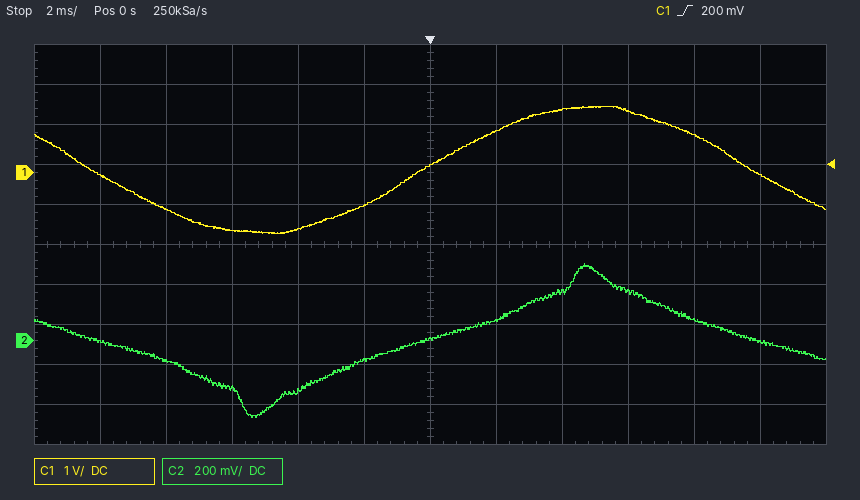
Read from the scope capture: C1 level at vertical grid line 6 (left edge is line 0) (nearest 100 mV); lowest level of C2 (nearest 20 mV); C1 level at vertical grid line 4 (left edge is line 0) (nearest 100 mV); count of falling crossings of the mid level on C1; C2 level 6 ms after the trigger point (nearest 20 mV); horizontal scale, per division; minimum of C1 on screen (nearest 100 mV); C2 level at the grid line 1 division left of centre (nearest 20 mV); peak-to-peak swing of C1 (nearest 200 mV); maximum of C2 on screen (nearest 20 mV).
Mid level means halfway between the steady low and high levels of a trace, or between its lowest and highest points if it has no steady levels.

200 mV
-380 mV
-1.4 V
2
240 mV
2 ms
-1.5 V
-100 mV
3.2 V
380 mV
